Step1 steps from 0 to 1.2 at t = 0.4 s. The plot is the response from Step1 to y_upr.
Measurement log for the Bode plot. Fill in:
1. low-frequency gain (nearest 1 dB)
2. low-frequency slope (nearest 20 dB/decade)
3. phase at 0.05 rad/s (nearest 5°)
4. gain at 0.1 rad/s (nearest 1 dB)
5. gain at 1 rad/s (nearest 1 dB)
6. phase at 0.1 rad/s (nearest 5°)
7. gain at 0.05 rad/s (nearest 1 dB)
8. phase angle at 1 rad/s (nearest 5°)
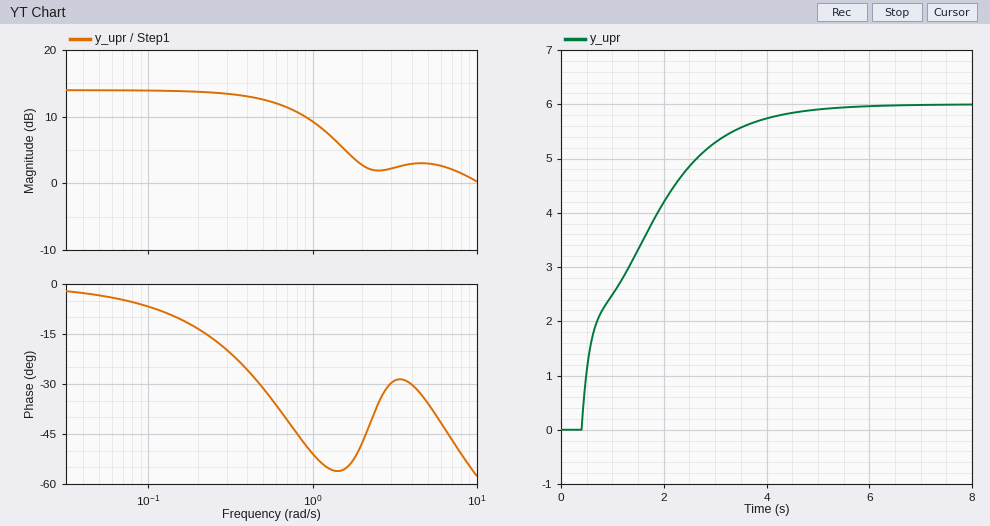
14 dB
0 dB/decade
-5°
14 dB
9 dB
-5°
14 dB
-50°
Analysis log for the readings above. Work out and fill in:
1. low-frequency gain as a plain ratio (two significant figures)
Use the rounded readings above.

5.0
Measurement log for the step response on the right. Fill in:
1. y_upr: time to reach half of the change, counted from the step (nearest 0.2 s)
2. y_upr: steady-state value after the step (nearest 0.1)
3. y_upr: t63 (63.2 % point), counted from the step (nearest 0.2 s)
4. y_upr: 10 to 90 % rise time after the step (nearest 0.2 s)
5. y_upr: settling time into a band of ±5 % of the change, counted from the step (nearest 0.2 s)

1.0 s
6.0
1.4 s
2.8 s
3.4 s
